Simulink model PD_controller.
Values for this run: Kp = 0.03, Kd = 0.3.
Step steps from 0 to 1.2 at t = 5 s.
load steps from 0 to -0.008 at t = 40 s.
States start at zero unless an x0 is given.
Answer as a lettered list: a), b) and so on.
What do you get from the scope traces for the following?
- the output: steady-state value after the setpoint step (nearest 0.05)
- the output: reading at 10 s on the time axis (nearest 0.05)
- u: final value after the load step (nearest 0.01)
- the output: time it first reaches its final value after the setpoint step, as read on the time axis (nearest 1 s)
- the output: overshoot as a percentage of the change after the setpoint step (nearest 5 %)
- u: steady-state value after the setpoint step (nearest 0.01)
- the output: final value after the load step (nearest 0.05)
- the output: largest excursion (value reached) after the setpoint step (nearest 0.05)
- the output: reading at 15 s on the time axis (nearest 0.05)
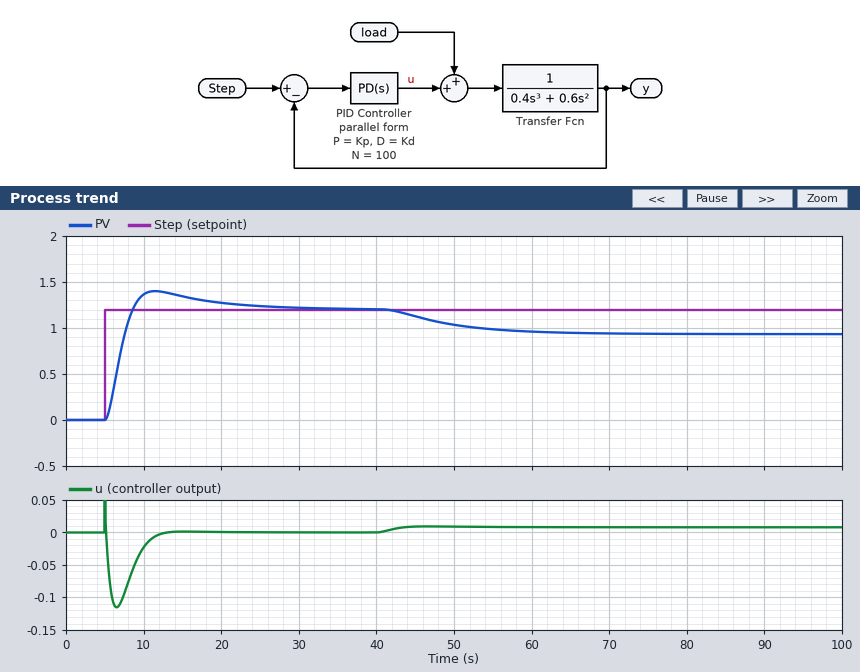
a) 1.20
b) 1.35
c) 0.01
d) 9 s
e) 15 %
f) 0.00
g) 0.95
h) 1.40
i) 1.35
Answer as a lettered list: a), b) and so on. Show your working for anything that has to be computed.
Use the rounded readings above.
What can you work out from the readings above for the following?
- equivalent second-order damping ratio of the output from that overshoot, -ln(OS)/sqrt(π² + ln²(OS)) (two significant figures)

a) ln(0.15) = -1.897; 1.897 / sqrt(9.870 + 3.599) = 0.52
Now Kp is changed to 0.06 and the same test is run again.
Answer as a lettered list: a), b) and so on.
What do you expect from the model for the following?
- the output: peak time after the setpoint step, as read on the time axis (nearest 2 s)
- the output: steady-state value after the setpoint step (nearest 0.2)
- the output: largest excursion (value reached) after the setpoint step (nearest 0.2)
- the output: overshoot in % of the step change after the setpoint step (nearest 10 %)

a) 10 s
b) 1.2
c) 1.6
d) 30 %
